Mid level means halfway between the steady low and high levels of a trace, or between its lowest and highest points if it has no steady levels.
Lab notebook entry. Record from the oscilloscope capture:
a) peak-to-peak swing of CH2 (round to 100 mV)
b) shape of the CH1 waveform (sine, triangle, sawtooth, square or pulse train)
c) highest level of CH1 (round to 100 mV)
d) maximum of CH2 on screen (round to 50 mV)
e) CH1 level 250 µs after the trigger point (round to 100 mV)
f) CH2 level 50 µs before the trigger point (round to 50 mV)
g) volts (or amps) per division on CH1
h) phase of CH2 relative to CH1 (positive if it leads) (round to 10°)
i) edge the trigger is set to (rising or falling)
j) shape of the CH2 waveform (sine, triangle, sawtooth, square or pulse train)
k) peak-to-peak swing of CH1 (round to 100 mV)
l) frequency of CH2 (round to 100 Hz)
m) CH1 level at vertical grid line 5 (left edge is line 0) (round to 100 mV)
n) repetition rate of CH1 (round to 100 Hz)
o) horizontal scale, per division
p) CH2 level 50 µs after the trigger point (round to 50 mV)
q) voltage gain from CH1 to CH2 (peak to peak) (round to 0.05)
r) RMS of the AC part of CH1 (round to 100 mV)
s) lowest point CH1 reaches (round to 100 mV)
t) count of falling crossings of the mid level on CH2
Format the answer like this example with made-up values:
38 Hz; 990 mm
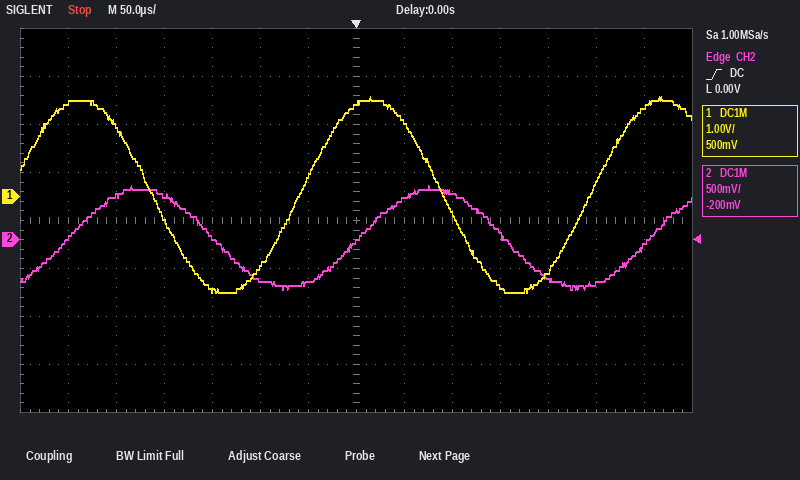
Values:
1.10 V; sine; 2.1 V; 550 mV; 300 mV; -450 mV; 1 V; -70°; rising; sine; 4.1 V; 3.3 kHz; -1.4 V; 3.3 kHz; 50 µs; 450 mV; 0.25; 1.4 V; -2.0 V; 2
